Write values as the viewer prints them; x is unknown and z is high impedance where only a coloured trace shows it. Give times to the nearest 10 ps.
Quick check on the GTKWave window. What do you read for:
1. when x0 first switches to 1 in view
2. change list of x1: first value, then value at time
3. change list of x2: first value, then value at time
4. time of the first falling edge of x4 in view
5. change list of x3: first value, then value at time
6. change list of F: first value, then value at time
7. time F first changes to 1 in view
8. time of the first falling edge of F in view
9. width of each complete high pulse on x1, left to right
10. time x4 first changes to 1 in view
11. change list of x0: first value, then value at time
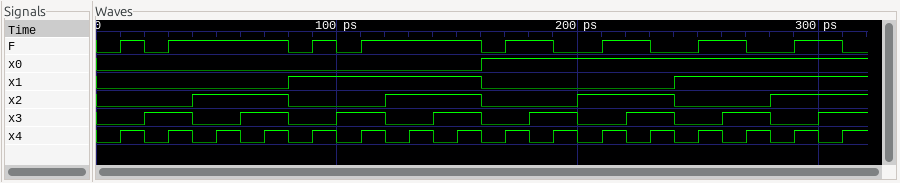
160 ps
0, 1 at 80 ps, 0 at 160 ps, 1 at 240 ps
0, 1 at 40 ps, 0 at 80 ps, 1 at 120 ps, 0 at 160 ps, 1 at 200 ps, 0 at 240 ps, 1 at 280 ps
20 ps
0, 1 at 20 ps, 0 at 40 ps, 1 at 60 ps, 0 at 80 ps, 1 at 100 ps, 0 at 120 ps, 1 at 140 ps, 0 at 160 ps, 1 at 180 ps, 0 at 200 ps, 1 at 220 ps, 0 at 240 ps, 1 at 260 ps, 0 at 280 ps, 1 at 300 ps
0, 1 at 10 ps, 0 at 20 ps, 1 at 30 ps, 0 at 80 ps, 1 at 90 ps, 0 at 100 ps, 1 at 110 ps, 0 at 160 ps, 1 at 170 ps, 0 at 190 ps, 1 at 210 ps, 0 at 230 ps, 1 at 250 ps, 0 at 270 ps, 1 at 290 ps, 0 at 310 ps
10 ps
20 ps
80 ps
10 ps
0, 1 at 160 ps
